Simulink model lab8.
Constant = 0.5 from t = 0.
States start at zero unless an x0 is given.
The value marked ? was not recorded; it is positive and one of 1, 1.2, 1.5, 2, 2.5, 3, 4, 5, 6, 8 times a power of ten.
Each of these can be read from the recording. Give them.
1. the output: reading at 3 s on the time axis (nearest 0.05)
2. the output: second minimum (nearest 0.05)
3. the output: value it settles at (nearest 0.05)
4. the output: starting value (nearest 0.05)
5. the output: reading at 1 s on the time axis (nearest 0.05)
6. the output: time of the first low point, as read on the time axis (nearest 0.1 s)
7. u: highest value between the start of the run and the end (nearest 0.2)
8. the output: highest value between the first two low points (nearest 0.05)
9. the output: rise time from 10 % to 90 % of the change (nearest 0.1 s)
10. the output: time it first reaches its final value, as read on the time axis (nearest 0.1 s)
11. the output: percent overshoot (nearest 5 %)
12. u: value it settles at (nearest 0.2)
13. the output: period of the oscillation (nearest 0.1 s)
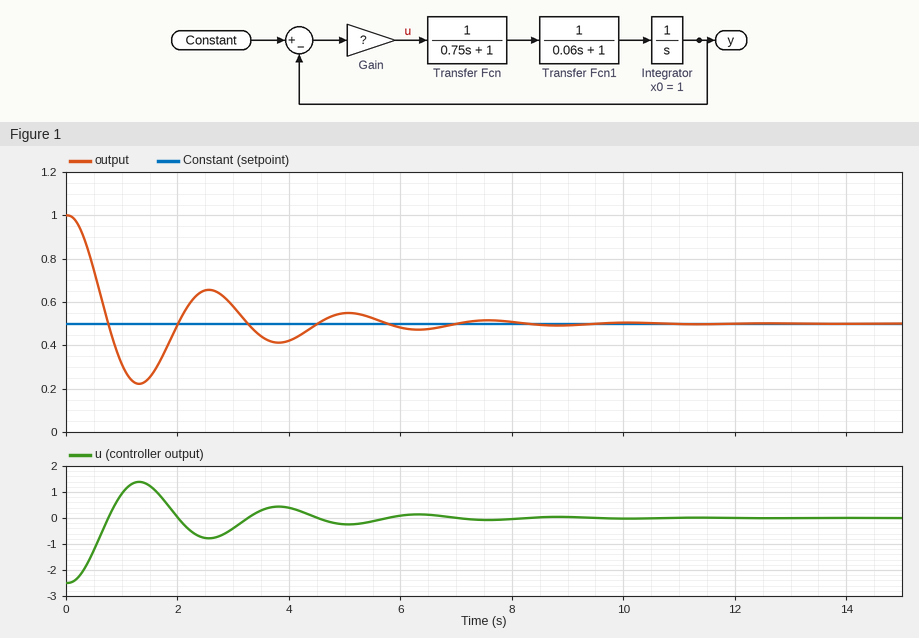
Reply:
0.60
0.40
0.50
1.00
0.30
1.3 s
1.4
0.65
0.5 s
0.8 s
55 %
0.0
2.5 s
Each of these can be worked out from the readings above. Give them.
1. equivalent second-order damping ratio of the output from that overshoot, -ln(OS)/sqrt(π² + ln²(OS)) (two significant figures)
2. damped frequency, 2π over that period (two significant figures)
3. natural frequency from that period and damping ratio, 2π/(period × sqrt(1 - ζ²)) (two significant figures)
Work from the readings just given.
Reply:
0.19
2.5 rad/s
2.6 rad/s
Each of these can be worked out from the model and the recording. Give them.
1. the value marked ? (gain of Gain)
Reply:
5
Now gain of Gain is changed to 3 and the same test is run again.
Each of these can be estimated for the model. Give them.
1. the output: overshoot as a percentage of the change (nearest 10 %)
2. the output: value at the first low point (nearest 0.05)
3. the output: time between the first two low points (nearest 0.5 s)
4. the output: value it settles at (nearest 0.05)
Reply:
40 %
0.30
3.5 s
0.50
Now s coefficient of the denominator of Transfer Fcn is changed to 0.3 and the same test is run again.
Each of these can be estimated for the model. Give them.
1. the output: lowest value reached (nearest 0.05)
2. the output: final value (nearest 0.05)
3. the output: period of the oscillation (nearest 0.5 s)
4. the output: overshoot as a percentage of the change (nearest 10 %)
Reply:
0.30
0.50
1.5 s
40 %
